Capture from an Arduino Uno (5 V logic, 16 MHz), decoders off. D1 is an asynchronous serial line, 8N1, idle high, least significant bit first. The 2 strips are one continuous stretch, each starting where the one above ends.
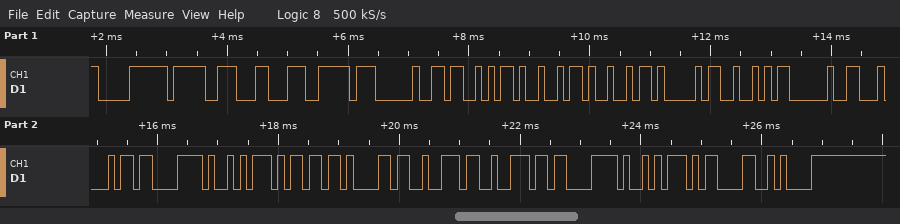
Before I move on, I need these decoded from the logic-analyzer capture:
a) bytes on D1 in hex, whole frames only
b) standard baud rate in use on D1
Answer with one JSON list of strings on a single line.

["F0 9F 8C BE 20 53 49 49 41 52 20 44 C3 A9 6D 61 72 72 C3 A9 0D 0A", "9600 baud"]
